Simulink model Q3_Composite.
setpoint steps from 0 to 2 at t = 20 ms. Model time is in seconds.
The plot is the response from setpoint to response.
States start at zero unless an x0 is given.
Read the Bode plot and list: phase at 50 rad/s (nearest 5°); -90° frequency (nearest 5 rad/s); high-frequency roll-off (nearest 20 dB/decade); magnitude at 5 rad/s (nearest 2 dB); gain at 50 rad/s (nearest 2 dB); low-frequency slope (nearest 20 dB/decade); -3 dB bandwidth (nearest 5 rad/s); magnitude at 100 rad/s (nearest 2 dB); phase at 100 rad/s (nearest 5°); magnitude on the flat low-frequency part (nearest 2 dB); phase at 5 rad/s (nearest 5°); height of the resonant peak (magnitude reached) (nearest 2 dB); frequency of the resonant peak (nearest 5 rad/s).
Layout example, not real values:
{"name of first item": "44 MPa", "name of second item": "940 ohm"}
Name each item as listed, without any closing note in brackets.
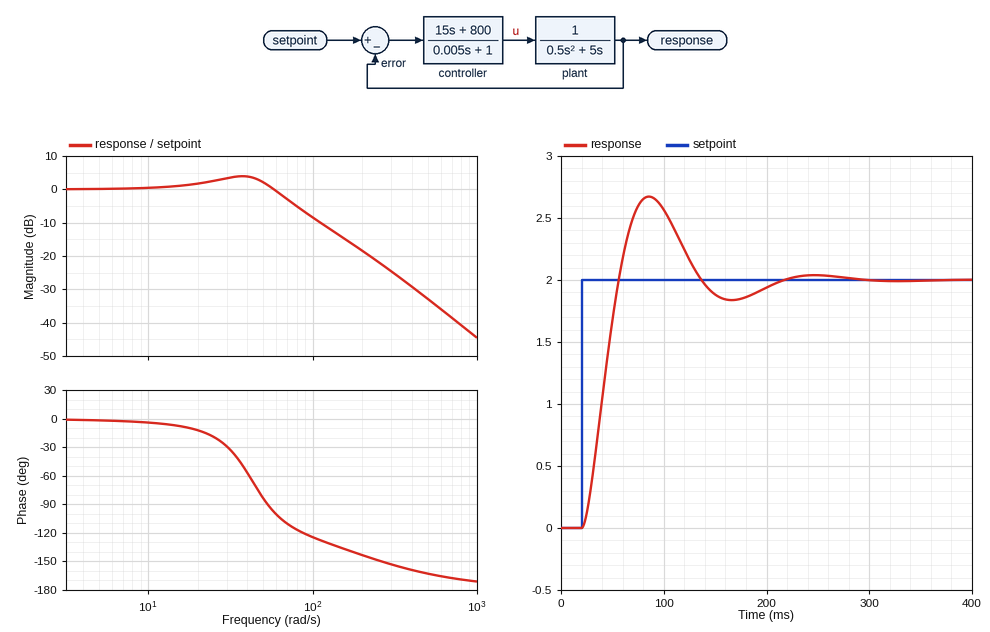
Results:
{"phase at 50 rad/s": "-85°", "-90° frequency": "55 rad/s", "high-frequency roll-off": "-40 dB/decade", "magnitude at 5 rad/s": "0 dB", "gain at 50 rad/s": "2 dB", "low-frequency slope": "0 dB/decade", "-3 dB bandwidth": "70 rad/s", "magnitude at 100 rad/s": "-8 dB", "phase at 100 rad/s": "-125°", "magnitude on the flat low-frequency part": "0 dB", "phase at 5 rad/s": "0°", "height of the resonant peak (magnitude reached)": "4 dB", "frequency of the resonant peak": "35 rad/s"}
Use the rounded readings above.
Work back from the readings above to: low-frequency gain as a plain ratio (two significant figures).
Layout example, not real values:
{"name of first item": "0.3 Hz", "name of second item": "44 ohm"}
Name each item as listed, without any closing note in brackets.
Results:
{"low-frequency gain as a plain ratio": "1.0"}
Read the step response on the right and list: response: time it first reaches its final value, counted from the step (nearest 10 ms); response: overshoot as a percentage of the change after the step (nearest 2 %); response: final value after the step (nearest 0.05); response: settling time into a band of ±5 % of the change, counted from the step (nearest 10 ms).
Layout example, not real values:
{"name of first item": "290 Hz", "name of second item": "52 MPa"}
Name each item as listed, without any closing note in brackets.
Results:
{"response: time it first reaches its final value, counted from the step": "40 ms", "response: overshoot as a percentage of the change after the step": "34 %", "response: final value after the step": "2.00", "response: settling time into a band of ±5 % of the change, counted from the step": "170 ms"}
